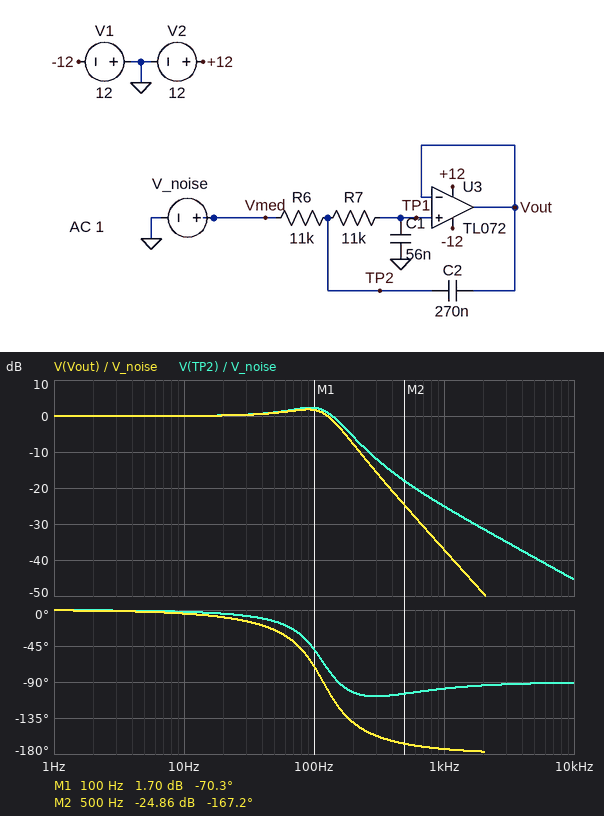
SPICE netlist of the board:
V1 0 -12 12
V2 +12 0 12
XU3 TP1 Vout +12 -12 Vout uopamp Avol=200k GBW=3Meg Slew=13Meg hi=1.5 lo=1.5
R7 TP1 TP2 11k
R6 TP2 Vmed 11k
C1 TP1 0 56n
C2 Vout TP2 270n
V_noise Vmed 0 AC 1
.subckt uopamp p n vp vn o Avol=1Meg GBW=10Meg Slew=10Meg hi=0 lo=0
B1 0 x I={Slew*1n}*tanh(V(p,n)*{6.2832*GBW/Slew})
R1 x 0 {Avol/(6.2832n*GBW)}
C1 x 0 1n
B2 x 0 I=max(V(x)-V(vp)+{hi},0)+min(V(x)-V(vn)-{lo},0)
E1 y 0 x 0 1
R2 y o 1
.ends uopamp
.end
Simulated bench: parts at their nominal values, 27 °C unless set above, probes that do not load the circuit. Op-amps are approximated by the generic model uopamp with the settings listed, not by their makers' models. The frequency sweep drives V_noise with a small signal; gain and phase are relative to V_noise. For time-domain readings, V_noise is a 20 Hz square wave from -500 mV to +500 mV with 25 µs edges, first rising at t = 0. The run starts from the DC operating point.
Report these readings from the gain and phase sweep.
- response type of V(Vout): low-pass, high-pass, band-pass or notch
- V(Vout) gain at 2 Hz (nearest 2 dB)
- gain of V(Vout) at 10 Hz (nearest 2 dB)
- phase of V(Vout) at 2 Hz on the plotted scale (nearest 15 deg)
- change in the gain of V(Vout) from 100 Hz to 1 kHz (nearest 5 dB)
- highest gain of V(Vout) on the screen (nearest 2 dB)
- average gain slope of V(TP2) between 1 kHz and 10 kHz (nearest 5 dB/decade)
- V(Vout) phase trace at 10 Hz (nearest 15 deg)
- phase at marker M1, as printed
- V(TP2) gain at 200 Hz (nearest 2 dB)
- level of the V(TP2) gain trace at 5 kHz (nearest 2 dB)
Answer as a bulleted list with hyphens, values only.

- low-pass
- 0 dB
- 0 dB
- 0 deg
- -40 dB
- 2 dB
- -20 dB/decade
- 0 deg
- -70.3 deg
- -6 dB
- -40 dB
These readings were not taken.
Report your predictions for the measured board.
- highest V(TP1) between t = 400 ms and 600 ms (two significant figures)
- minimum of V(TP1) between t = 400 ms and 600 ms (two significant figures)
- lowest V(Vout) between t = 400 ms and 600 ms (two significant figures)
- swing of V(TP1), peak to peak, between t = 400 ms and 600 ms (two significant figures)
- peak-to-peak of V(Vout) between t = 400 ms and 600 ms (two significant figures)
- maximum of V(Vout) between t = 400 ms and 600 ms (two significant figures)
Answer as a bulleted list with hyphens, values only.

- 700 mV
- -700 mV
- -700 mV
- 1.4 V
- 1.4 V
- 700 mV
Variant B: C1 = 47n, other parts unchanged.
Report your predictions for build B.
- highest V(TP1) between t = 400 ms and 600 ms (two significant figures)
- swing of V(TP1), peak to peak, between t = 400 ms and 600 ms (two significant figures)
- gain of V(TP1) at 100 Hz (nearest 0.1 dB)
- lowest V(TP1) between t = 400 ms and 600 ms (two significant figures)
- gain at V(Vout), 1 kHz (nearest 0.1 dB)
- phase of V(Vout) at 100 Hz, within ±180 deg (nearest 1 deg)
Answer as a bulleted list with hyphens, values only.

- 740 mV
- 1.5 V
- 2.4 dB
- -740 mV
- -35.6 dB
- -59 deg
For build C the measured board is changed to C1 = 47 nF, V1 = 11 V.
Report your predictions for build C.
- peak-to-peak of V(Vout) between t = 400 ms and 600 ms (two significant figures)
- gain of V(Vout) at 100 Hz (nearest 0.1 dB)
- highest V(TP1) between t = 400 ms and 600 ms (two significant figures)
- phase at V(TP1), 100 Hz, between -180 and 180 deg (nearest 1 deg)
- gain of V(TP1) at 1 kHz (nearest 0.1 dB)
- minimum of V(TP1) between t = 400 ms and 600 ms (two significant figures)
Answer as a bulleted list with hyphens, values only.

- 1.5 V
- 2.4 dB
- 740 mV
- -59 deg
- -35.6 dB
- -740 mV
